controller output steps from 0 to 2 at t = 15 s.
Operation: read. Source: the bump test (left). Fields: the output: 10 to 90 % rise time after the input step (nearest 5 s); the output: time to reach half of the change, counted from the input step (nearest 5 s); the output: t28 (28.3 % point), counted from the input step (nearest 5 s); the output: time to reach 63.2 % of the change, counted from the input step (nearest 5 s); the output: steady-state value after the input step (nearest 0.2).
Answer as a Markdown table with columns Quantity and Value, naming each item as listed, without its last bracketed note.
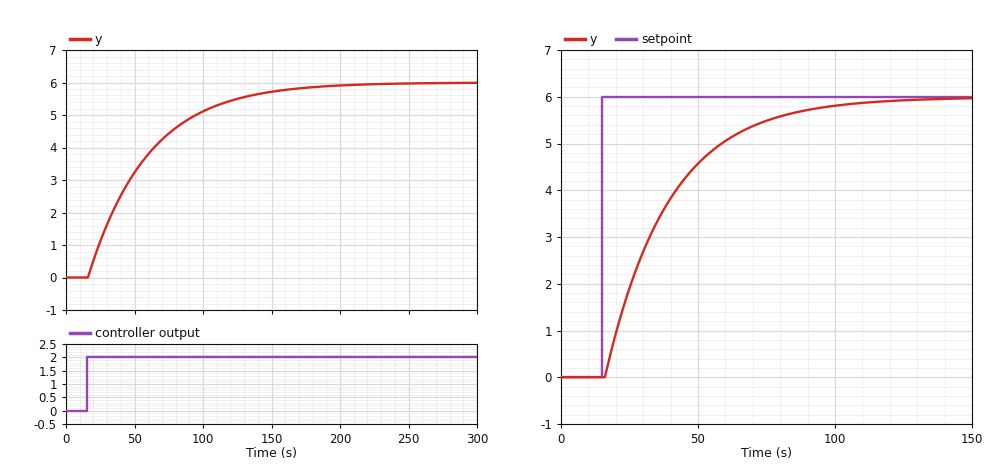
| Quantity | Value |
|---|---|
| the output: 10 to 90 % rise time after the input step | 95 s |
| the output: time to reach half of the change, counted from the input step | 30 s |
| the output: t28 (28.3 % point), counted from the input step | 15 s |
| the output: time to reach 63.2 % of the change, counted from the input step | 45 s |
| the output: steady-state value after the input step | 6.0 |
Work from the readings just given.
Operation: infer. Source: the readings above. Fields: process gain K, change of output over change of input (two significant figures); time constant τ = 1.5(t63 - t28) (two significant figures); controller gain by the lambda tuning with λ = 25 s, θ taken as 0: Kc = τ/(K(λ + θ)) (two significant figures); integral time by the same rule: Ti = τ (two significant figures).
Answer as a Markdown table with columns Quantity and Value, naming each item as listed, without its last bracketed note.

| Quantity | Value |
|---|---|
| process gain K, change of output over change of input | 3.0 |
| time constant τ = 1.5(t63 - t28) | 45 s |
| controller gain by the lambda tuning with λ = 25 s, θ taken as 0: Kc = τ/(K(λ + θ)) | 0.60 |
| integral time by the same rule: Ti = τ | 45 s |
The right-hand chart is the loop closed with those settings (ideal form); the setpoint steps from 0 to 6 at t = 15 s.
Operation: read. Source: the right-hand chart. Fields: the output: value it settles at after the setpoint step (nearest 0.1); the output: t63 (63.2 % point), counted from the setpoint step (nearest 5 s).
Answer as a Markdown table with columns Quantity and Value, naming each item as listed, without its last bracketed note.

| Quantity | Value |
|---|---|
| the output: value it settles at after the setpoint step | 6.0 |
| the output: t63 (63.2 % point), counted from the setpoint step | 25 s |
